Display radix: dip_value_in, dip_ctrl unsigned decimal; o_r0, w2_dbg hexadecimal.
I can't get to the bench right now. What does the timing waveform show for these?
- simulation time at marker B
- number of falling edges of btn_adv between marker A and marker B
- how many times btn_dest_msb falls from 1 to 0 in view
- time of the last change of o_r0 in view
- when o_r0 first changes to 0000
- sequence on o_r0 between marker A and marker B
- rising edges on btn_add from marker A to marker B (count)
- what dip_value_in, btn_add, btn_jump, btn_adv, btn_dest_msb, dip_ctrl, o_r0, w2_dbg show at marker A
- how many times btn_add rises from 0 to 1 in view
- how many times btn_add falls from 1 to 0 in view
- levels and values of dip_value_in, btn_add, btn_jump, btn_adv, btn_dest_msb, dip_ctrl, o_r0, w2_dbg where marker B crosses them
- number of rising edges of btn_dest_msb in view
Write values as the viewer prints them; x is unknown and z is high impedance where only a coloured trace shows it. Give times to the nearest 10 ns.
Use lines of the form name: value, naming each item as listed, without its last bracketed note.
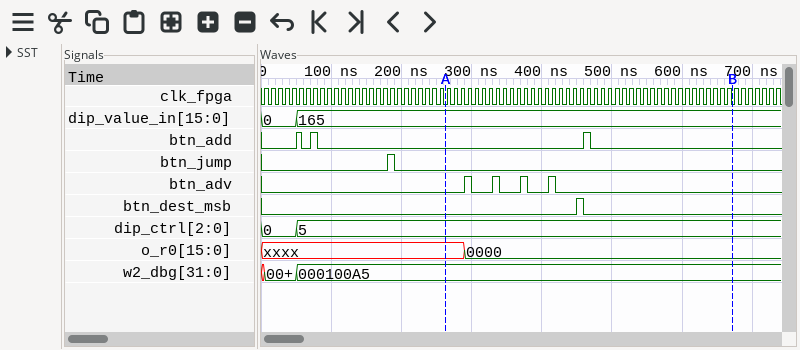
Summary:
simulation time at marker B: 670 ns
number of falling edges of btn_adv between marker A and marker B: 4
how many times btn_dest_msb falls from 1 to 0 in view: 1
time of the last change of o_r0 in view: 290 ns
when o_r0 first changes to 0000: 290 ns
sequence on o_r0 between marker A and marker B: xxxx, 0000
rising edges on btn_add from marker A to marker B: 1
what dip_value_in, btn_add, btn_jump, btn_adv, btn_dest_msb, dip_ctrl, o_r0, w2_dbg show at marker A: dip_value_in=165, btn_add=0, btn_jump=0, btn_adv=0, btn_dest_msb=0, dip_ctrl=5, o_r0=xxxx, w2_dbg=000100A5
how many times btn_add rises from 0 to 1 in view: 3
how many times btn_add falls from 1 to 0 in view: 3
levels and values of dip_value_in, btn_add, btn_jump, btn_adv, btn_dest_msb, dip_ctrl, o_r0, w2_dbg where marker B crosses them: dip_value_in=165, btn_add=0, btn_jump=0, btn_adv=0, btn_dest_msb=0, dip_ctrl=5, o_r0=0000, w2_dbg=000100A5
number of rising edges of btn_dest_msb in view: 1
